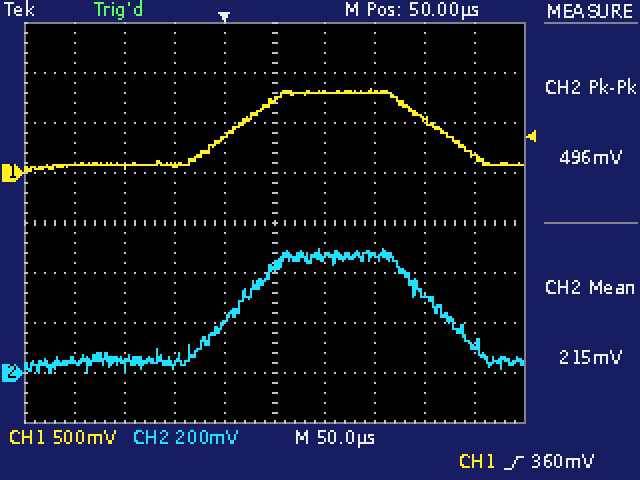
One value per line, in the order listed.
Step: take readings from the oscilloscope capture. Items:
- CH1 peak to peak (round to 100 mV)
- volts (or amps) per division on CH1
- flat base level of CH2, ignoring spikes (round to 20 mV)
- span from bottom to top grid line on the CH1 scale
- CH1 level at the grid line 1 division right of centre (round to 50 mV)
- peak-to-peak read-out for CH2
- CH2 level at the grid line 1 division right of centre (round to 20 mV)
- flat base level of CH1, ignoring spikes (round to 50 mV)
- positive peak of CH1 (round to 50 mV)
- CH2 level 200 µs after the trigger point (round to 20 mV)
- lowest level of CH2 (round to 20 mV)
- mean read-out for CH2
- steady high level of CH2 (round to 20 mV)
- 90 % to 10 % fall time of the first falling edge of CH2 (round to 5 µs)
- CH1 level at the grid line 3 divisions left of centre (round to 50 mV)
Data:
800 mV
500 mV
40 mV
4 V
800 mV
496 mV
460 mV
100 mV
850 mV
320 mV
0 mV
215 mV
460 mV
80 µs
50 mV
